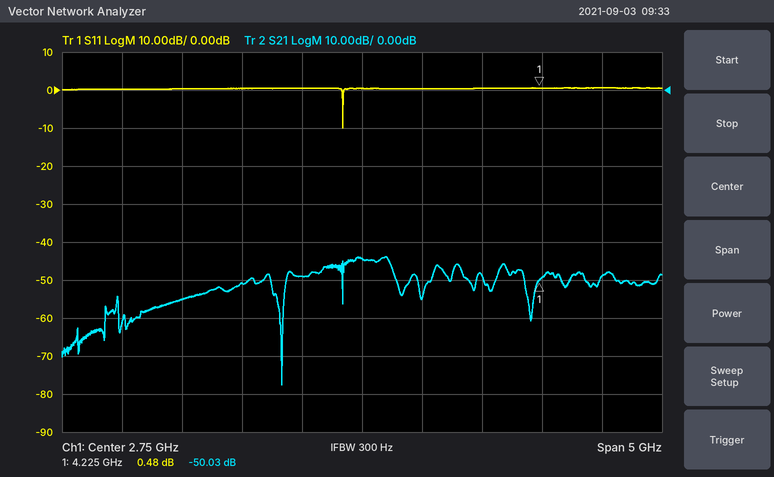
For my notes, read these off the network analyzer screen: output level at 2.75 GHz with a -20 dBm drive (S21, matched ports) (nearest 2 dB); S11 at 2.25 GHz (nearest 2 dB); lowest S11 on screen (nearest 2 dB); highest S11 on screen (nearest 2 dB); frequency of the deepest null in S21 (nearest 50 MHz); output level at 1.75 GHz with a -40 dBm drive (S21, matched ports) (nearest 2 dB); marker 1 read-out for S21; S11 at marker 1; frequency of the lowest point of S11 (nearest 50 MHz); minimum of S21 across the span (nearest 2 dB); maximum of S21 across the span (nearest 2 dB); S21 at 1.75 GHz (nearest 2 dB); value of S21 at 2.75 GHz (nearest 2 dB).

-64 dBm
0 dB
-10 dB
0 dB
2.10 GHz
-90 dBm
-50.03 dB
0.48 dB
2.60 GHz
-78 dB
-44 dB
-50 dB
-44 dB
